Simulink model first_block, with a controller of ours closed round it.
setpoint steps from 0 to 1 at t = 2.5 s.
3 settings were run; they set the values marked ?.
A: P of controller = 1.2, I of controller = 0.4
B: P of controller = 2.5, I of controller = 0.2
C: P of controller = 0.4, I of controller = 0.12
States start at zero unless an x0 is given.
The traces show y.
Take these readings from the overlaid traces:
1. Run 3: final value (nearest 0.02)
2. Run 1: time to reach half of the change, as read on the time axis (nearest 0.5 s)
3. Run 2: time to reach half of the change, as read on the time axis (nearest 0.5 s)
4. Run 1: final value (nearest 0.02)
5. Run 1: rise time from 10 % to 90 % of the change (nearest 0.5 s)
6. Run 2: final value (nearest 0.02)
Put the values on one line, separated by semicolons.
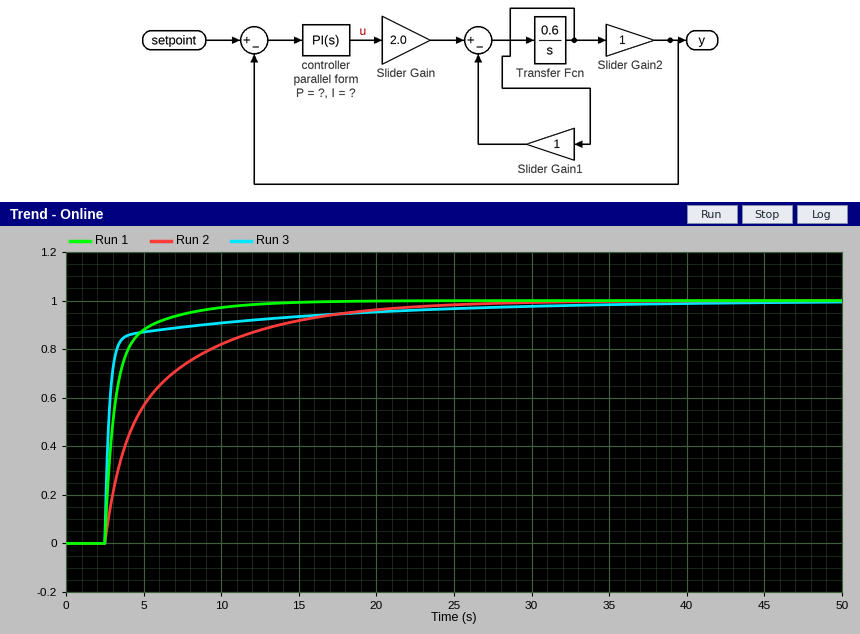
1.00; 3.0 s; 4.5 s; 1.00; 3.0 s; 1.00
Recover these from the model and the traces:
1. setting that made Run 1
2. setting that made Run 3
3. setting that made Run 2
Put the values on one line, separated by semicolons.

A; B; C
